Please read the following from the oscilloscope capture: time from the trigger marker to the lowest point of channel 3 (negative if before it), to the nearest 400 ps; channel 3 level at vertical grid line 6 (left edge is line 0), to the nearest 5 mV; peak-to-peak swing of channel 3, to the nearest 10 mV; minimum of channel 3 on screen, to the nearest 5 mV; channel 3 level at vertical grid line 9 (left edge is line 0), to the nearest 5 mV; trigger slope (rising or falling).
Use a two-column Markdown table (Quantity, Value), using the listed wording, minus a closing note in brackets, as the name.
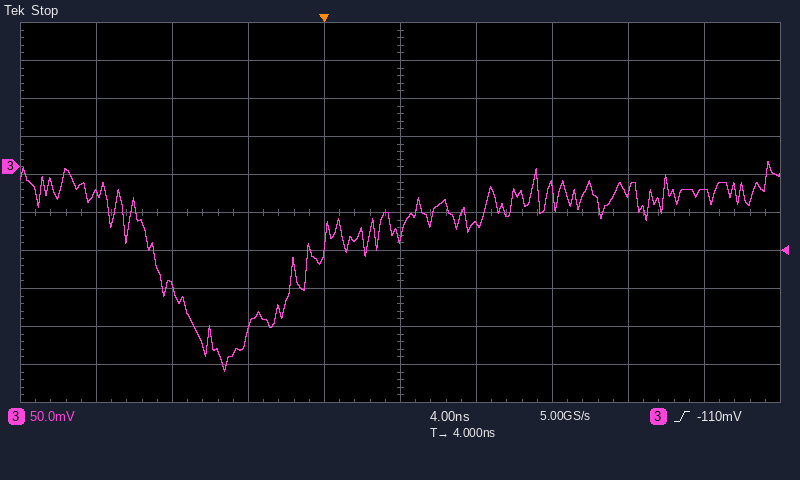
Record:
| Quantity | Value |
|---|---|
| time from the trigger marker to the lowest point of channel 3 (negative if before it), to the nearest 400 ps | -5.2 ns |
| channel 3 level at vertical grid line 6 (left edge is line 0), to the nearest 5 mV | -75 mV |
| peak-to-peak swing of channel 3, to the nearest 10 mV | 280 mV |
| minimum of channel 3 on screen, to the nearest 5 mV | -270 mV |
| channel 3 level at vertical grid line 9 (left edge is line 0), to the nearest 5 mV | -30 mV |
| trigger slope | rising |
